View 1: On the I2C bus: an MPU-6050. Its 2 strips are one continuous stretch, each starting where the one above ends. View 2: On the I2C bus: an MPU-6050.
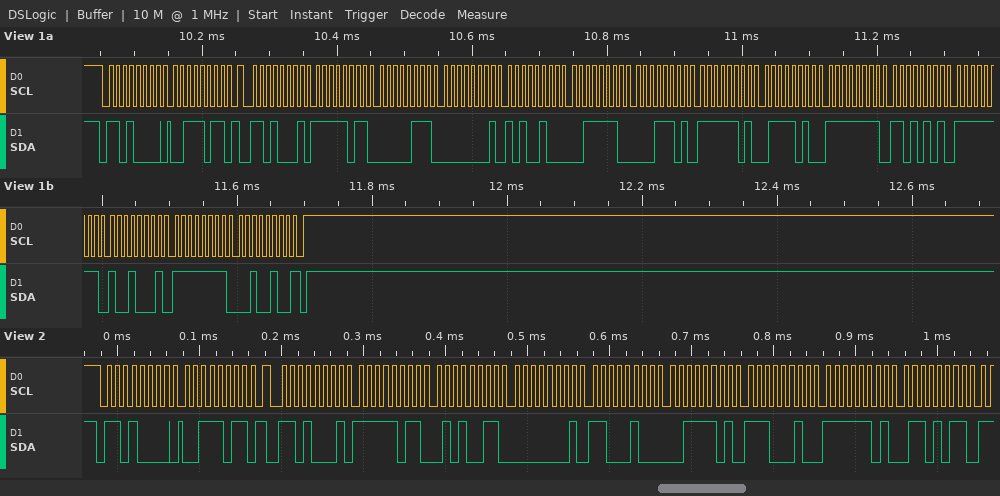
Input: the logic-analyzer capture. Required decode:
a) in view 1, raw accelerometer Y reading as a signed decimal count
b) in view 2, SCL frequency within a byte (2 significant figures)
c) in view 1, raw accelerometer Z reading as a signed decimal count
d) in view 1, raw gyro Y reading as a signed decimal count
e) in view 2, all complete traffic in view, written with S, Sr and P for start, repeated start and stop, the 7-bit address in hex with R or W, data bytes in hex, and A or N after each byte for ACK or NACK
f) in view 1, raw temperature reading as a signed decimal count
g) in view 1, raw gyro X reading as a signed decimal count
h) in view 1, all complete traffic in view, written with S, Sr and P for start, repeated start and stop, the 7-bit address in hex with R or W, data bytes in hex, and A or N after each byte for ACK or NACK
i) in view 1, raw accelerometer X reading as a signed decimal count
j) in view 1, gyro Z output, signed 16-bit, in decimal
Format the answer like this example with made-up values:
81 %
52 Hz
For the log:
420
100 kHz
15901
-111
S 68W A 3B A Sr 68R A FB A 53 A 01 A C4 A 3D A E2 A FD A 6B A
-646
-43
S 68W A 3B A Sr 68R A FB A 07 A 01 A A4 A 3E A 1D A FD A 7A A FF A D5 A FF A 91 A FF A 24 N P
-1273
-220
